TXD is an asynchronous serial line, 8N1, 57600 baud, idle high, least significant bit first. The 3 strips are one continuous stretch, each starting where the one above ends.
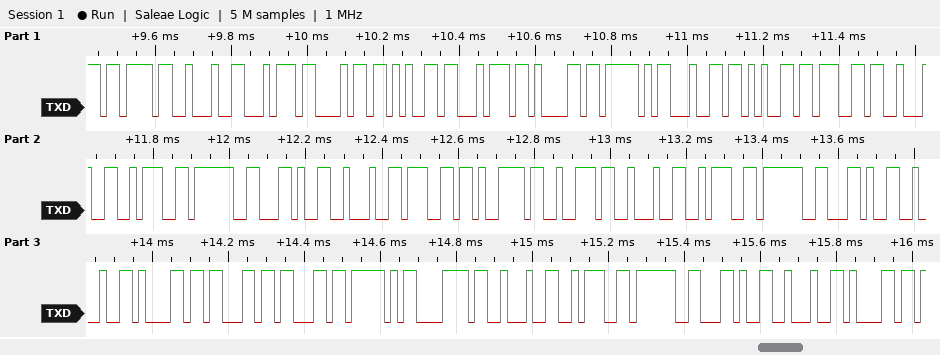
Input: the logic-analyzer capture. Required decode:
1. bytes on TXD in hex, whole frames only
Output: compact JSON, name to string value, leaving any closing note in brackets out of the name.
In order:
{"bytes on TXD in hex, whole frames only": "0x7B 0x22 0x74 0x68 0x65 0x74 0x61 0x5F 0x64 0x65 0x67 0x22 0x3A 0x3F 0x2C 0x22 0x67 0x79 0x72 0x22 0x3A 0x3F 0x2C 0x22 0x61 0x63 0x63 0x5F 0x78 0x22 0x3A 0x3F 0x2C 0x22 0x61"}
